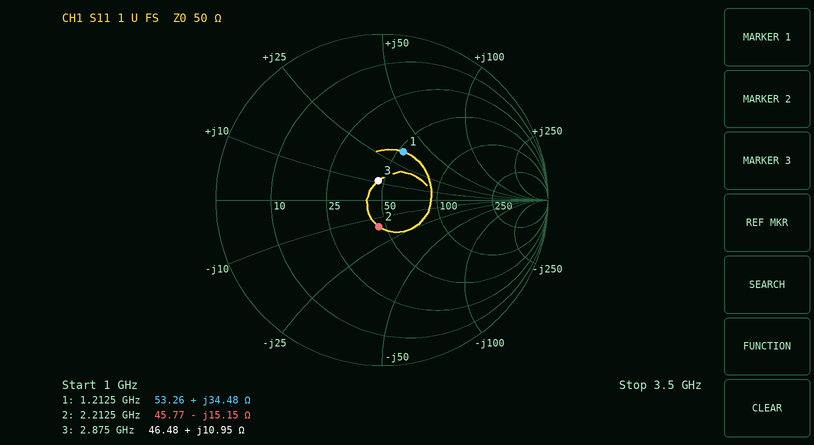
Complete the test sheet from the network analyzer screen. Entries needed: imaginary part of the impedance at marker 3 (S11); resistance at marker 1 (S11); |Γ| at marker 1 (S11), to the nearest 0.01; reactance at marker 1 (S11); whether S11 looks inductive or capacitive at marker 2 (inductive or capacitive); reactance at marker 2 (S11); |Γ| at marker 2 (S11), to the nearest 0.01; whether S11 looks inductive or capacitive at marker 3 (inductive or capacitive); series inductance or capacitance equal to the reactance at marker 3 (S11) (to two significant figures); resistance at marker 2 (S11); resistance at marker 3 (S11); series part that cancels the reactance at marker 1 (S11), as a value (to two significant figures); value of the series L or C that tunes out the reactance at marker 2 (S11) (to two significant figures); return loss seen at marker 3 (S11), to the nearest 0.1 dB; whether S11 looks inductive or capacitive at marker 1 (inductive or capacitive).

+10.95 Ω
53.26 Ω
0.32
+34.48 Ω
capacitive
-15.15 Ω
0.16
inductive
610 pH
45.77 Ω
46.48 Ω
3.8 pF
1.1 nH
18.5 dB
inductive
